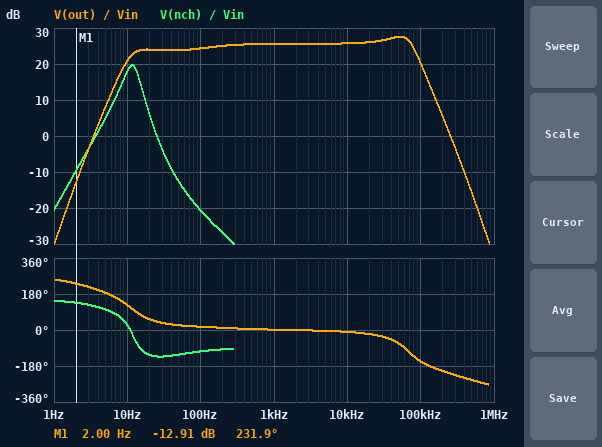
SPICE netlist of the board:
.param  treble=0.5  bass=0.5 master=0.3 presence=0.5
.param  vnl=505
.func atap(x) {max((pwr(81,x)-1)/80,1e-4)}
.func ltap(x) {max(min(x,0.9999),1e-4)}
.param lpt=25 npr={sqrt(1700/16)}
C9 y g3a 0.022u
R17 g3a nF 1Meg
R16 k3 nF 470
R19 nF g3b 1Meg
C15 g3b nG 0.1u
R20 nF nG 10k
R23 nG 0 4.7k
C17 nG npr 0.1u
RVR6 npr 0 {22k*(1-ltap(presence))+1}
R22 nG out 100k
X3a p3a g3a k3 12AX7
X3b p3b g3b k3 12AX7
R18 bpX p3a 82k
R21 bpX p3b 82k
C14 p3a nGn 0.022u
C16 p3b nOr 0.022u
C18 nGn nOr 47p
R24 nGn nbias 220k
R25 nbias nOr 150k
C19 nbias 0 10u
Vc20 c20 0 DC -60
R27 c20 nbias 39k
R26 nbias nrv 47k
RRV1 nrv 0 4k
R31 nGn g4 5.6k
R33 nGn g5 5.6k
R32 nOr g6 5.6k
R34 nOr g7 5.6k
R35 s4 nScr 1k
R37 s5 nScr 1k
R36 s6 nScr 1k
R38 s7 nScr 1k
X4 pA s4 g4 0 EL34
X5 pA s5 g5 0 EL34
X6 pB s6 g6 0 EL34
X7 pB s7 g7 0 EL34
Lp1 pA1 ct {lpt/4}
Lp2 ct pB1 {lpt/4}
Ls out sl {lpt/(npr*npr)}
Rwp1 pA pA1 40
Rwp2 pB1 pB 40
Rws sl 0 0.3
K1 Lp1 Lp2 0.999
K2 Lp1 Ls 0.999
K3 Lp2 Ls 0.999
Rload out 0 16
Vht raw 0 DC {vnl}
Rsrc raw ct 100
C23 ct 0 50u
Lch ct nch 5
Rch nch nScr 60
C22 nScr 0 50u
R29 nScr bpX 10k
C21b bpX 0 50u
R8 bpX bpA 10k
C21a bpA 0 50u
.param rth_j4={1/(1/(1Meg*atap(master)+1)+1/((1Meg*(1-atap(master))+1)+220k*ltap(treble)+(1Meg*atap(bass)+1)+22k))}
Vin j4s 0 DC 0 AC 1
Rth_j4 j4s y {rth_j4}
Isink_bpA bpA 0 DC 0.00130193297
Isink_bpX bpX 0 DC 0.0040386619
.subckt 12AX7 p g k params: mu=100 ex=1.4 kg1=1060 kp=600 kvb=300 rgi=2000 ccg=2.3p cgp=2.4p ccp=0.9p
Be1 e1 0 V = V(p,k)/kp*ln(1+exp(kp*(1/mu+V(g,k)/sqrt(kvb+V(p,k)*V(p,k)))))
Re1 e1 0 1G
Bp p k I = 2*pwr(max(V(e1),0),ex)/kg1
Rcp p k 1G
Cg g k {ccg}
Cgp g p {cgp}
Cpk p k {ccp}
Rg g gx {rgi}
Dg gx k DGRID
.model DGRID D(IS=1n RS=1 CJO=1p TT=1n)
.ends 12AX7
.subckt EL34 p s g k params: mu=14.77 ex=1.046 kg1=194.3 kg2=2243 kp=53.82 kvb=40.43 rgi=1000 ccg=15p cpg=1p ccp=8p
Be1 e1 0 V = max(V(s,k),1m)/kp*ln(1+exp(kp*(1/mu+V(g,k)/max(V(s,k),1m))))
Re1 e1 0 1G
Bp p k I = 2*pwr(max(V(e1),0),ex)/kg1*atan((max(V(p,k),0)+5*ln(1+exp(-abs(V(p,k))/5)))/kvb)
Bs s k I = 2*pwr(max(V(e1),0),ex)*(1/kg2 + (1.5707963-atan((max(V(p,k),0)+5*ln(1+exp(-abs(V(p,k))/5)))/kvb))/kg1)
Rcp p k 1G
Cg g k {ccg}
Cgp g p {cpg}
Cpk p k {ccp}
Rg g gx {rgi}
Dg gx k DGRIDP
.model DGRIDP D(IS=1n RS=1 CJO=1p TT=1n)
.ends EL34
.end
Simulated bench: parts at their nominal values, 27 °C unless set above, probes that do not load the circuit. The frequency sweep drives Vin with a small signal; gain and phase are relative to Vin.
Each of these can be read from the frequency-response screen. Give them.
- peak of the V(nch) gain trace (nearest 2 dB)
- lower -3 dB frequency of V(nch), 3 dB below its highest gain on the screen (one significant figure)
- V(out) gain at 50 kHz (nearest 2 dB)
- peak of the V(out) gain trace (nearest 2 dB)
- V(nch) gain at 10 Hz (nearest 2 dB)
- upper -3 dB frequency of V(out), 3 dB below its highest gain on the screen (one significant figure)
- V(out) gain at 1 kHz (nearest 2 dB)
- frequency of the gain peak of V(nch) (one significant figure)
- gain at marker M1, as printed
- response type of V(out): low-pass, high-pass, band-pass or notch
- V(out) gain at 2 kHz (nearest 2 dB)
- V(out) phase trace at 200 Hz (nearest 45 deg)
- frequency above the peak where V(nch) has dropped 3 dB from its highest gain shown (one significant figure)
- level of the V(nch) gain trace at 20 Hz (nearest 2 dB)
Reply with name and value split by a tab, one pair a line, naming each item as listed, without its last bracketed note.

peak of the V(nch) gain trace	20 dB
lower -3 dB frequency of V(nch), 3 dB below its highest gain on the screen	9 Hz
V(out) gain at 50 kHz	28 dB
peak of the V(out) gain trace	28 dB
V(nch) gain at 10 Hz	18 dB
upper -3 dB frequency of V(out), 3 dB below its highest gain on the screen	80 kHz
V(out) gain at 1 kHz	26 dB
frequency of the gain peak of V(nch)	10 Hz
gain at marker M1, as printed	-12.91 dB
response type of V(out): low-pass, high-pass, band-pass or notch	band-pass
V(out) gain at 2 kHz	26 dB
V(out) phase trace at 200 Hz	0 deg
frequency above the peak where V(nch) has dropped 3 dB from its highest gain shown	10 Hz
level of the V(nch) gain trace at 20 Hz	6 dB
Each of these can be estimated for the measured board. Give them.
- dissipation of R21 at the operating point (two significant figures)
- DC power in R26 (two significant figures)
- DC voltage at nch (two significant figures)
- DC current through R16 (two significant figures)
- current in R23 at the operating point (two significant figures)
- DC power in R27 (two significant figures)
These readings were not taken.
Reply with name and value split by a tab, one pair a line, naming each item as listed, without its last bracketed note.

dissipation of R21 at the operating point	180 mW
DC power in R26	21 mW
DC voltage at nch	470 V
DC current through R16	3.0 mA
current in R23 at the operating point	2.8 mA
DC power in R27	17 mW
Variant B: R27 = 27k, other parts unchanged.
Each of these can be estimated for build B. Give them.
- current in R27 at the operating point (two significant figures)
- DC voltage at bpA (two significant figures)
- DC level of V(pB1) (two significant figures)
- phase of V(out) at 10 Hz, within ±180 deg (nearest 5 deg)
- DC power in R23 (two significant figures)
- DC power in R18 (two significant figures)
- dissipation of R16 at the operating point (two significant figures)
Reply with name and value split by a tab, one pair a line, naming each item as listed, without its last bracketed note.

current in R27 at the operating point	770 µA
DC voltage at bpA	380 V
DC level of V(pB1)	480 V
phase of V(out) at 10 Hz, within ±180 deg	130 deg
DC power in R23	40 mW
DC power in R18	190 mW
dissipation of R16 at the operating point	4.4 mW
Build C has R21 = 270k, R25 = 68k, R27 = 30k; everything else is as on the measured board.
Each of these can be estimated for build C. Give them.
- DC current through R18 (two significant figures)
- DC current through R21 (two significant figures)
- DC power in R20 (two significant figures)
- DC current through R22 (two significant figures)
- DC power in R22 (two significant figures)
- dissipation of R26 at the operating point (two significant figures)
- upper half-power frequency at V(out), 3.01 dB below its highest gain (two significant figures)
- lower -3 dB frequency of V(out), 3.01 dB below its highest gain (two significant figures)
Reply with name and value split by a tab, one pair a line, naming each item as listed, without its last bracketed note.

DC current through R18	1.8 mA
DC current through R21	730 µA
DC power in R20	64 mW
DC current through R22	110 µA
DC power in R22	1.3 mW
dissipation of R26 at the operating point	26 mW
upper half-power frequency at V(out), 3.01 dB below its highest gain	80 kHz
lower -3 dB frequency of V(out), 3.01 dB below its highest gain	45 Hz
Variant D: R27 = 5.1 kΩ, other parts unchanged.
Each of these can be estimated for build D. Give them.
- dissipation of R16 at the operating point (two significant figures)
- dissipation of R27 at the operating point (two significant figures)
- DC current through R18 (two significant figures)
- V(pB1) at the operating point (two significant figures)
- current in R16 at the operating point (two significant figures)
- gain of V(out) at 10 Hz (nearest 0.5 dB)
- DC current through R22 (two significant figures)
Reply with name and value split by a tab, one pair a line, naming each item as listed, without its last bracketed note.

dissipation of R16 at the operating point	4.8 mW
dissipation of R27 at the operating point	5.8 mW
DC current through R18	1.6 mA
V(pB1) at the operating point	500 V
current in R16 at the operating point	3.2 mA
gain of V(out) at 10 Hz	6.0 dB
DC current through R22	140 µA
